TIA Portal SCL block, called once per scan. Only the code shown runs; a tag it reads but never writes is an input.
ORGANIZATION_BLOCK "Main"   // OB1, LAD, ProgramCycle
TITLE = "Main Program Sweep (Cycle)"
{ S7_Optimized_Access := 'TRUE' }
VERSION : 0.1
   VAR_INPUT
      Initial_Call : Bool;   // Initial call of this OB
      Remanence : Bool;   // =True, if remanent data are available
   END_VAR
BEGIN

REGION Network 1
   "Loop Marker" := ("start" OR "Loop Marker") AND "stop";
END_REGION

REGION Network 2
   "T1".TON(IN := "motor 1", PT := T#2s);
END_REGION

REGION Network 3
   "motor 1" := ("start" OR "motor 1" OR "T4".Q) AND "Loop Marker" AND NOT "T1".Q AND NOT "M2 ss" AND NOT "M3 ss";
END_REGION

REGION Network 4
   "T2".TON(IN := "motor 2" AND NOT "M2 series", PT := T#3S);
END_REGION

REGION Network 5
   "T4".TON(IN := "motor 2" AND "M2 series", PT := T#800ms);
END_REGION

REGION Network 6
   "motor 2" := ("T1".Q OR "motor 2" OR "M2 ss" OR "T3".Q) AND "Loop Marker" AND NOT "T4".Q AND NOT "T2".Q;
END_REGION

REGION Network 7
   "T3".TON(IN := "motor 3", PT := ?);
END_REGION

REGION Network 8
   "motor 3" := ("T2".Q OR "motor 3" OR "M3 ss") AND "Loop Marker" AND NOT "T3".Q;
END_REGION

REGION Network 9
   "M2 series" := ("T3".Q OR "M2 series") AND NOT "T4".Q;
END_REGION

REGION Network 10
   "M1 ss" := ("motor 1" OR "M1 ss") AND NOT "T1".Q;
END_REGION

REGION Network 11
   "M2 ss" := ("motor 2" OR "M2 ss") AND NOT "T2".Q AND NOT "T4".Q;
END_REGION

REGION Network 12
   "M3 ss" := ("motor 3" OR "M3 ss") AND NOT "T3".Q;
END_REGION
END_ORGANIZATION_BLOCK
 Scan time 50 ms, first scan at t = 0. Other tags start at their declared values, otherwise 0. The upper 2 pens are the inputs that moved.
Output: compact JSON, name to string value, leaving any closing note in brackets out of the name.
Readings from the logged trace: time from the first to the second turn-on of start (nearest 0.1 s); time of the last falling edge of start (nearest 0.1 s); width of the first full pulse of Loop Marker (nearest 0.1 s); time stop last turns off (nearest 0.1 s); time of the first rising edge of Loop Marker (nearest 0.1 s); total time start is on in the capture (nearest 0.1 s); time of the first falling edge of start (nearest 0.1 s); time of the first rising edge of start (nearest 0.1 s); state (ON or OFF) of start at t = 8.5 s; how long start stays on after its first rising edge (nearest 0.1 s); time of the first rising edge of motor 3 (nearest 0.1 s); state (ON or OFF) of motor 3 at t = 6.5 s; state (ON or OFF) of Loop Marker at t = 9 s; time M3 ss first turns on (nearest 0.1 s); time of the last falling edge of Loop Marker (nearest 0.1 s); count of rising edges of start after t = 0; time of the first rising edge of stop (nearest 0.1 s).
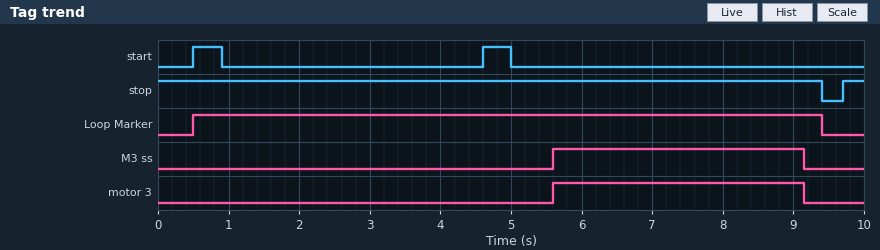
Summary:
{"time from the first to the second turn-on of start": "4.1 s", "time of the last falling edge of start": "5.0 s", "width of the first full pulse of Loop Marker": "8.9 s", "time stop last turns off": "9.4 s", "time of the first rising edge of Loop Marker": "0.5 s", "total time start is on in the capture": "0.8 s", "time of the first falling edge of start": "0.9 s", "time of the first rising edge of start": "0.5 s", "state (ON or OFF) of start at t = 8.5 s": "OFF", "how long start stays on after its first rising edge": "0.4 s", "time of the first rising edge of motor 3": "5.6 s", "state (ON or OFF) of motor 3 at t = 6.5 s": "ON", "state (ON or OFF) of Loop Marker at t = 9 s": "ON", "time M3 ss first turns on": "5.6 s", "time of the last falling edge of Loop Marker": "9.4 s", "count of rising edges of start after t = 0": "2", "time of the first rising edge of stop": "9.7 s"}
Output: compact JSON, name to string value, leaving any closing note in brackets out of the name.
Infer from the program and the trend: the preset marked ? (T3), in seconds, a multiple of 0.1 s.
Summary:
{"the preset marked ? (T3), in seconds, a multiple of 0.1 s": "3.5 s"}
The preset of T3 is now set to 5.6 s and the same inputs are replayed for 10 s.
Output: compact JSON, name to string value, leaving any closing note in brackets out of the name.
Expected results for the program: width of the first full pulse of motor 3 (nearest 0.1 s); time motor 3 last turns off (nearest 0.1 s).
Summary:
{"width of the first full pulse of motor 3": "3.8 s", "time motor 3 last turns off": "9.4 s"}
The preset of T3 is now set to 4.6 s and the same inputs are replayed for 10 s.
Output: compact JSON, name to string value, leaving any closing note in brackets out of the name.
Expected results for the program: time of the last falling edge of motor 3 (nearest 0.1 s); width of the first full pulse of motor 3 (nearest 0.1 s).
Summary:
{"time of the last falling edge of motor 3": "9.4 s", "width of the first full pulse of motor 3": "3.8 s"}
